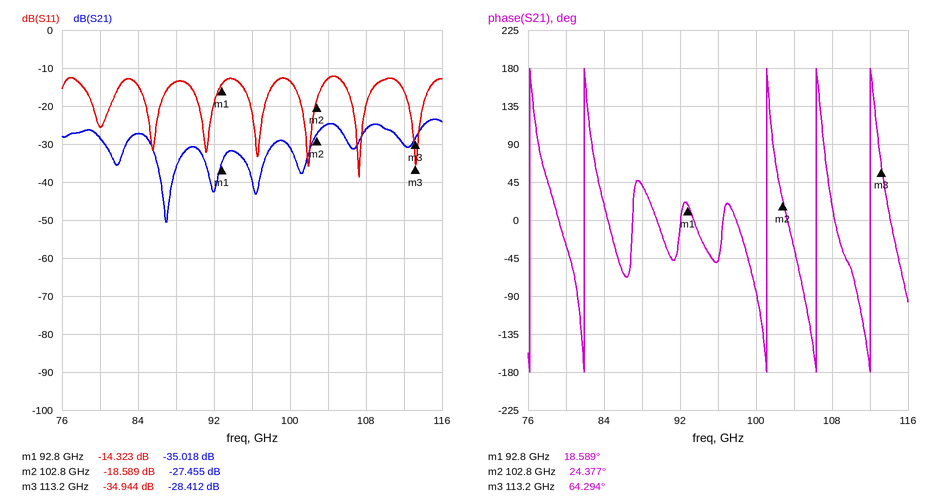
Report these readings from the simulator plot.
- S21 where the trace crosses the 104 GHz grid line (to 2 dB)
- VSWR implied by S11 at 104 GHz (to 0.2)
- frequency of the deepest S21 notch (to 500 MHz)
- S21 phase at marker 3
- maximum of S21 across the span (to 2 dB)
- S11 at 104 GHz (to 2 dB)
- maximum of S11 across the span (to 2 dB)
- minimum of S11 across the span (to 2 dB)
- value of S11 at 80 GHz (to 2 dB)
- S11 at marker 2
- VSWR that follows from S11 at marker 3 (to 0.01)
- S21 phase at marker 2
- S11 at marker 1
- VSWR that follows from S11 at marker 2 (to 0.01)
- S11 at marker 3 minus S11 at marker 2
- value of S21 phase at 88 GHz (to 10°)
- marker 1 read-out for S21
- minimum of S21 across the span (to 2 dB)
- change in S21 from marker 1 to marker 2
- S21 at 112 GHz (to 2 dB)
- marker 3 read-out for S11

-24 dB
1.6
87.0 GHz
64.294°
-24 dB
-12 dB
-12 dB
-38 dB
-26 dB
-18.589 dB
1.04
24.377°
-14.323 dB
1.27
-16.355 dB
40°
-35.018 dB
-50 dB
7.563 dB
-30 dB
-34.944 dB
